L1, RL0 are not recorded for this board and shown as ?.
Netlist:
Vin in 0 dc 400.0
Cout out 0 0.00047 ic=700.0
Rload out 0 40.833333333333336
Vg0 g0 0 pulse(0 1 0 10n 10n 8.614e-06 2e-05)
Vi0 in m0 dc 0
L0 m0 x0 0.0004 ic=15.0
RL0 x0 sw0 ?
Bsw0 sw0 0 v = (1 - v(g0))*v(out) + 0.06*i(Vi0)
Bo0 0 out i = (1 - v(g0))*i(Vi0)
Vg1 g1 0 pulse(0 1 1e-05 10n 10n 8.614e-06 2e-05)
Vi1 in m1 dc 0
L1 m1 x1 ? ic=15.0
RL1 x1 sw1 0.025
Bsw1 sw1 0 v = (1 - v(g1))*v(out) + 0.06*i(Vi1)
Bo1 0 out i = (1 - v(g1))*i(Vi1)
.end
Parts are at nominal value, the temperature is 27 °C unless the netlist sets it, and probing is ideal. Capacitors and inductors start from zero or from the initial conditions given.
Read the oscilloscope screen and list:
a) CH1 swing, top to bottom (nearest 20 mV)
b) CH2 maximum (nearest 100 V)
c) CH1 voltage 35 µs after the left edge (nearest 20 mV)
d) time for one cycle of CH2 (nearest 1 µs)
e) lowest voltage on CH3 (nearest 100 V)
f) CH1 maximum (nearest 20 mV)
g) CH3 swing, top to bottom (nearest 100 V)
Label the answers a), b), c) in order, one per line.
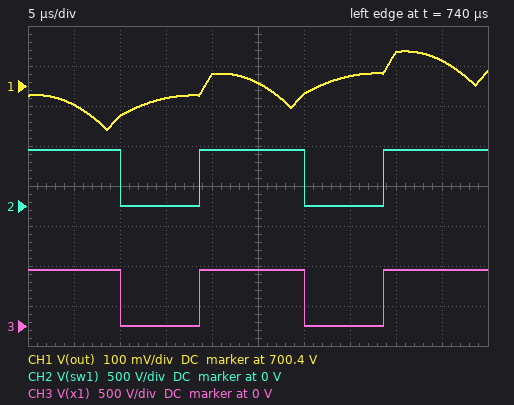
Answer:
a) 200 mV
b) 700 V
c) 700.42 V
d) 20 µs
e) 0 V
f) 700.48 V
g) 700 V
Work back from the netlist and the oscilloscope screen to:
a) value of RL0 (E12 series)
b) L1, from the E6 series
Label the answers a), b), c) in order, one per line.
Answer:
a) 0.022 Ω
b) 220 µH
